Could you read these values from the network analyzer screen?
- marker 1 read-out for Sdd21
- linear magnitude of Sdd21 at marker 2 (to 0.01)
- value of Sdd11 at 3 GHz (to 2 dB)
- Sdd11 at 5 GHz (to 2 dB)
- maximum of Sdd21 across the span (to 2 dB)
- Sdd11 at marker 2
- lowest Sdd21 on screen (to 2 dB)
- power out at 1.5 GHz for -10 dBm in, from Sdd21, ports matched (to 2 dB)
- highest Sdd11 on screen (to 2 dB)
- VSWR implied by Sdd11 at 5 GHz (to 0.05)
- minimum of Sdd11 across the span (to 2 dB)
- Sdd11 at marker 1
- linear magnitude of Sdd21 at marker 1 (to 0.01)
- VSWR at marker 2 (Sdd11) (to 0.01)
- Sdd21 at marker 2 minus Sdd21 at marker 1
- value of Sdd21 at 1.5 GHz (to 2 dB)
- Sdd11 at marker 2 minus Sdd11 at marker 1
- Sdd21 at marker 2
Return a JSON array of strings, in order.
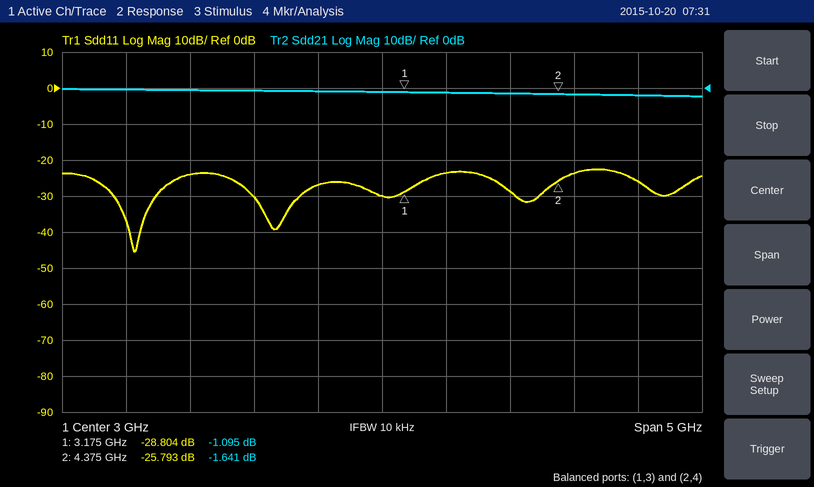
["-1.095 dB", "0.83", "-30 dB", "-26 dB", "0 dB", "-25.793 dB", "-2 dB", "-10 dBm", "-22 dB", "1.10", "-46 dB", "-28.804 dB", "0.88", "1.11", "-0.546 dB", "0 dB", "3.011 dB", "-1.641 dB"]
